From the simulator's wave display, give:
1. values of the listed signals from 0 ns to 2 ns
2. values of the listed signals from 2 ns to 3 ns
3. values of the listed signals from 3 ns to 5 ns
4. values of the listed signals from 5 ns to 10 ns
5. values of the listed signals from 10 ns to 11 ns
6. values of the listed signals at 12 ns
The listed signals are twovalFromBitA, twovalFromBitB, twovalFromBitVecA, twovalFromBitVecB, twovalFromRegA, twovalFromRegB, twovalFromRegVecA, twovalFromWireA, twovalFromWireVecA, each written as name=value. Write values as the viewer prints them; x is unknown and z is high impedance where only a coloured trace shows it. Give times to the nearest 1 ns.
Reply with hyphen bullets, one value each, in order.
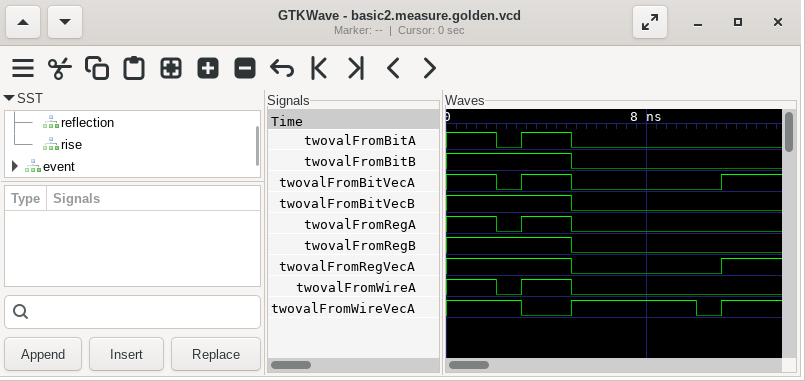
- twovalFromBitA=1, twovalFromBitB=1, twovalFromBitVecA=1, twovalFromBitVecB=1, twovalFromRegA=1, twovalFromRegB=1, twovalFromRegVecA=1, twovalFromWireA=1, twovalFromWireVecA=1
- twovalFromBitA=0, twovalFromBitB=1, twovalFromBitVecA=0, twovalFromBitVecB=1, twovalFromRegA=0, twovalFromRegB=1, twovalFromRegVecA=1, twovalFromWireA=0, twovalFromWireVecA=1
- twovalFromBitA=1, twovalFromBitB=1, twovalFromBitVecA=1, twovalFromBitVecB=1, twovalFromRegA=1, twovalFromRegB=1, twovalFromRegVecA=1, twovalFromWireA=1, twovalFromWireVecA=0
- twovalFromBitA=0, twovalFromBitB=0, twovalFromBitVecA=0, twovalFromBitVecB=0, twovalFromRegA=0, twovalFromRegB=0, twovalFromRegVecA=0, twovalFromWireA=0, twovalFromWireVecA=1
- twovalFromBitA=0, twovalFromBitB=0, twovalFromBitVecA=0, twovalFromBitVecB=0, twovalFromRegA=0, twovalFromRegB=0, twovalFromRegVecA=0, twovalFromWireA=0, twovalFromWireVecA=0
- twovalFromBitA=0, twovalFromBitB=0, twovalFromBitVecA=1, twovalFromBitVecB=0, twovalFromRegA=0, twovalFromRegB=0, twovalFromRegVecA=1, twovalFromWireA=0, twovalFromWireVecA=1
